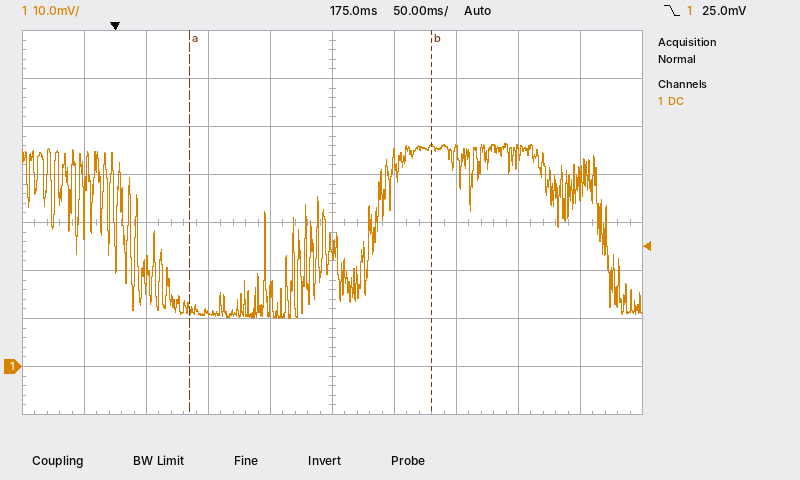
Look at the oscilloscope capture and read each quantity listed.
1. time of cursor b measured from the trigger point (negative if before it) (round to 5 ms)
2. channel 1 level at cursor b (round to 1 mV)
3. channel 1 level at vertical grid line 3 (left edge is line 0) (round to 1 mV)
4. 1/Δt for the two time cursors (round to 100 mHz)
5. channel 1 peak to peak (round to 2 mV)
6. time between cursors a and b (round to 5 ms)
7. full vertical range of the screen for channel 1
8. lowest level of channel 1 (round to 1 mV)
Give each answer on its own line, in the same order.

+255 ms
46 mV
11 mV
5.1 Hz
36 mV
195 ms
80 mV
10 mV
